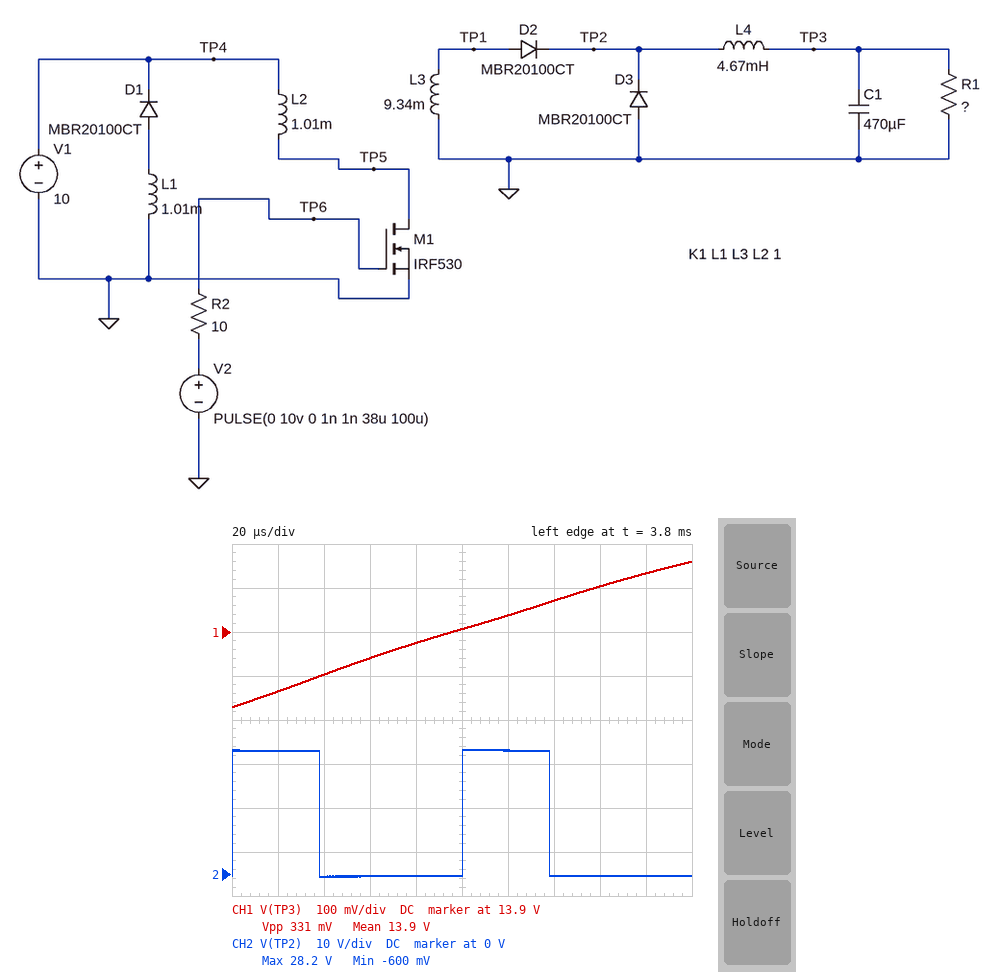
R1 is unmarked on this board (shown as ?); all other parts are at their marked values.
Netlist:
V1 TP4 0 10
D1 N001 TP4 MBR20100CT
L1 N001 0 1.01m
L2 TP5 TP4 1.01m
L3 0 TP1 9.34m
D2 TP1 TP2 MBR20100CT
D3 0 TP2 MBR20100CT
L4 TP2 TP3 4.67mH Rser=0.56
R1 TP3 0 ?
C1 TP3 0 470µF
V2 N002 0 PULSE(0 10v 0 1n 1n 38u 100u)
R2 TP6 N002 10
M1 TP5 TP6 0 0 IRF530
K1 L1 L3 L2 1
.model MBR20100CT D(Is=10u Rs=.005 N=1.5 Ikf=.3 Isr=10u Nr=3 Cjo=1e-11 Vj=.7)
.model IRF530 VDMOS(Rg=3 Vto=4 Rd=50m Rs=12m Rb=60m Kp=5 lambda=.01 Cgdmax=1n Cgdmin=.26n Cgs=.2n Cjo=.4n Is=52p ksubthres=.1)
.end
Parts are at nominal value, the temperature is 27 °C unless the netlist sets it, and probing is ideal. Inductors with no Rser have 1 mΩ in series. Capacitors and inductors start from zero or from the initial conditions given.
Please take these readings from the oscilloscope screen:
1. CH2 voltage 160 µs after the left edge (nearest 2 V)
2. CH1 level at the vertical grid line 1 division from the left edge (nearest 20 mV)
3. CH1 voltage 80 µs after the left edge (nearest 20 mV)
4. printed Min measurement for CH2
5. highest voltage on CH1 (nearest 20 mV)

0 V
13.76 V
13.88 V
-600 mV
14.06 V
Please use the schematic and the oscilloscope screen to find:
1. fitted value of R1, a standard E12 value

12 Ω
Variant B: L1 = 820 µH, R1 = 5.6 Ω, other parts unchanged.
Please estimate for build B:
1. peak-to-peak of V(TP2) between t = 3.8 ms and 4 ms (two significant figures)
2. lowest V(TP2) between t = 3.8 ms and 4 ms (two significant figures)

28 V
-590 mV
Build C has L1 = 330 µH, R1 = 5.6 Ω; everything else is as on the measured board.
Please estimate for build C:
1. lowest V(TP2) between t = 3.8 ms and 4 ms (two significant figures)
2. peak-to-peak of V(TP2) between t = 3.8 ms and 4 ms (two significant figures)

-590 mV
28 V
